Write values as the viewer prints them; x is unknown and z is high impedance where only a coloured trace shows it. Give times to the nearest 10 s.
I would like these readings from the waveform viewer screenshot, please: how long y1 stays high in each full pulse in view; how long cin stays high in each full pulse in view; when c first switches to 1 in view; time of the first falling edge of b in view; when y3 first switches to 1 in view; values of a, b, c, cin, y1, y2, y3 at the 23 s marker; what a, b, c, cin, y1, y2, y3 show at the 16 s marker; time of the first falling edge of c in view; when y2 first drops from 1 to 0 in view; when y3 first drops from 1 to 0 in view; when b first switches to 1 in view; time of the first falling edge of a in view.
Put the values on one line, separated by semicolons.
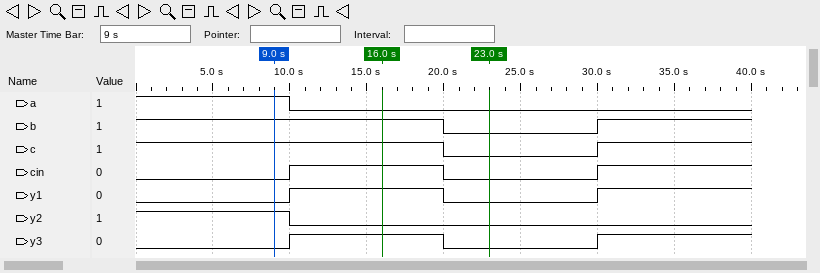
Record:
10 s; 10 s; 30 s; 20 s; 10 s; a=0, b=0, c=0, cin=0, y1=0, y2=0, y3=0; a=0, b=1, c=1, cin=1, y1=1, y2=0, y3=1; 20 s; 10 s; 20 s; 30 s; 10 s
